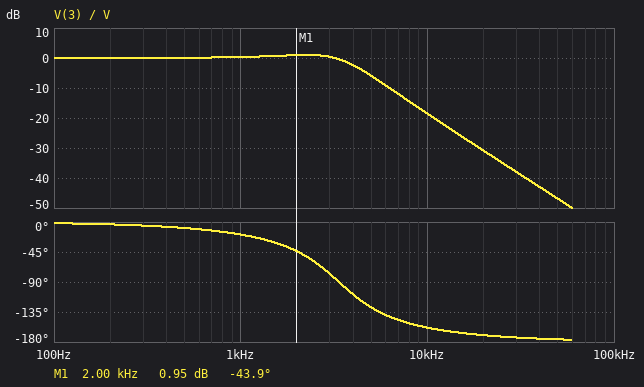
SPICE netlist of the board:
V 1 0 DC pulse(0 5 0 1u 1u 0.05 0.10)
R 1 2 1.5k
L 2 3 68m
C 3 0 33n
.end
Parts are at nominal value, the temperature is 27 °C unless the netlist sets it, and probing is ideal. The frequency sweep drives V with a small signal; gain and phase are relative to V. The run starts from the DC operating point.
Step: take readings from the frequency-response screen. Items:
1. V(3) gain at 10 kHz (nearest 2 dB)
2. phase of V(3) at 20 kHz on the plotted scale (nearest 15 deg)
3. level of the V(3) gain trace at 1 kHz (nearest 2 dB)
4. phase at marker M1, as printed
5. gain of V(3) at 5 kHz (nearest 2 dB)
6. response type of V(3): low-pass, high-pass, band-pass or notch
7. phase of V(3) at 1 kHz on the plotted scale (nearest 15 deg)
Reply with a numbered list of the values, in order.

1. -18 dB
2. -165 deg
3. 0 dB
4. -43.9 deg
5. -6 dB
6. low-pass
7. -15 deg
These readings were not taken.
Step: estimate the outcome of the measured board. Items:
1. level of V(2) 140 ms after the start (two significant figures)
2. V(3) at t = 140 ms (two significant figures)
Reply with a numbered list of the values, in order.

1. 5.0 V
2. 5.0 V
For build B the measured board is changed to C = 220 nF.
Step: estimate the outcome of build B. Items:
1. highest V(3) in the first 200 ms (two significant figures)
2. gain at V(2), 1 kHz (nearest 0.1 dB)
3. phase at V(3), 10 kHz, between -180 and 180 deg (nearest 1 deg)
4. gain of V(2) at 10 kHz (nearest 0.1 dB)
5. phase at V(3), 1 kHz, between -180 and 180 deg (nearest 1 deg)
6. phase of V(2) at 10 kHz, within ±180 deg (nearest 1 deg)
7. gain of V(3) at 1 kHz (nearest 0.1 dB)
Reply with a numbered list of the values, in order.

1. 5.0 V
2. -14.3 dB
3. -160 deg
4. -0.5 dB
5. -79 deg
6. 20 deg
7. -6.5 dB
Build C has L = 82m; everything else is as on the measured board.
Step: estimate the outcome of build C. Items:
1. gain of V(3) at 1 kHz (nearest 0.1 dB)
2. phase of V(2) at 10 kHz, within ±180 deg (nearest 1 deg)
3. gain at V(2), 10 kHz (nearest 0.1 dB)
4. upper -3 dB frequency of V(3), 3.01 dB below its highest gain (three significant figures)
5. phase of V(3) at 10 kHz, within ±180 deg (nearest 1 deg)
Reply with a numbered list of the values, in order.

1. 0.5 dB
2. 18 deg
3. -0.4 dB
4. 3.60 kHz
5. -162 deg
